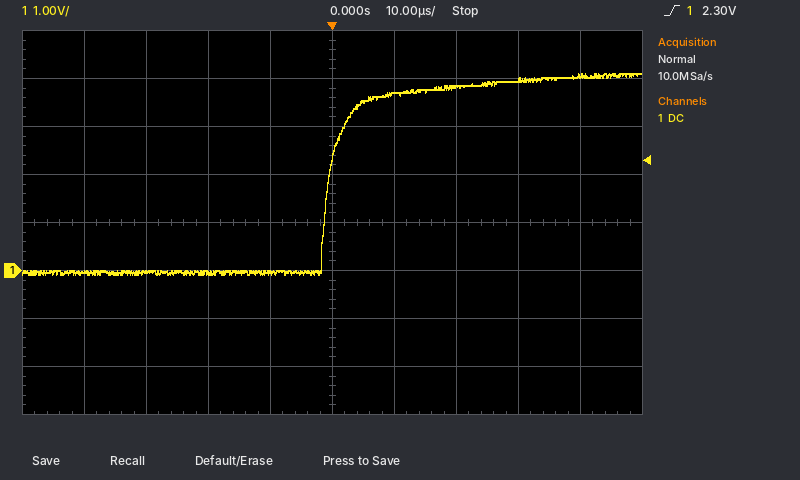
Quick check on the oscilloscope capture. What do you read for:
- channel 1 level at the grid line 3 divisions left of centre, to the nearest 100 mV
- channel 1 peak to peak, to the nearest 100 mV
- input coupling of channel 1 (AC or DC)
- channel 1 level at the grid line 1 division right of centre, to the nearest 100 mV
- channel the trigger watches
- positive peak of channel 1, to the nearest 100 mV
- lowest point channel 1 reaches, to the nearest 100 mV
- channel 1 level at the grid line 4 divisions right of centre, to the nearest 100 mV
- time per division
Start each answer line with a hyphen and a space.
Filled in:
- 0.0 V
- 4.2 V
- DC
- 3.7 V
- channel 1
- 4.1 V
- -100 mV
- 4.1 V
- 10 µs
